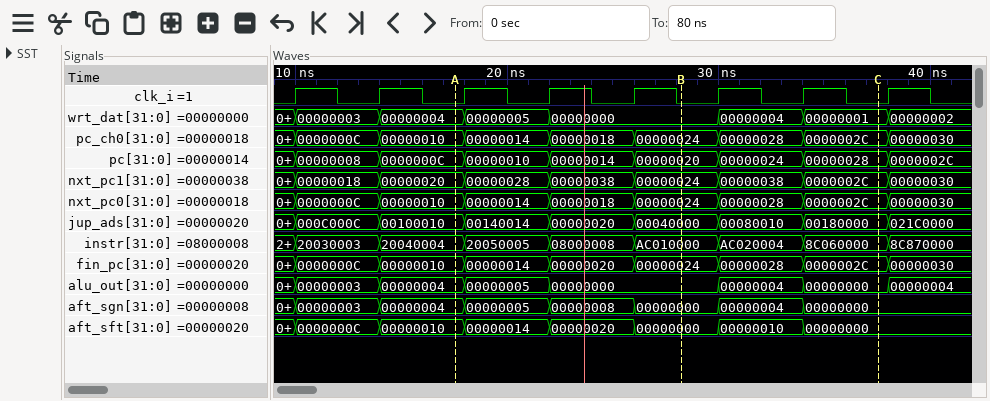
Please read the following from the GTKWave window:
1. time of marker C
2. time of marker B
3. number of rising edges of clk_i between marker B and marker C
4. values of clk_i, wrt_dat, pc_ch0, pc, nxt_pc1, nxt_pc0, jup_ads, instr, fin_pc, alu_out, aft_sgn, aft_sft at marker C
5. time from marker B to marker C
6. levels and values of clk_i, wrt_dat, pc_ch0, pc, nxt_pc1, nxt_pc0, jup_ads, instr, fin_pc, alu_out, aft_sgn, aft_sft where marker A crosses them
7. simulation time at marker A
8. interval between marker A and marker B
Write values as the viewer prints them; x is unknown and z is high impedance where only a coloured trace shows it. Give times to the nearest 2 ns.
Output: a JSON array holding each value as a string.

["38 ns", "28 ns", "2", "clk_i=0, wrt_dat=00000001, pc_ch0=0000002C, pc=00000028, nxt_pc1=0000002C, nxt_pc0=0000002C, jup_ads=00180000, instr=8C060000, fin_pc=0000002C, alu_out=00000000, aft_sgn=00000000, aft_sft=00000000", "10 ns", "clk_i=0, wrt_dat=00000004, pc_ch0=00000010, pc=0000000C, nxt_pc1=00000020, nxt_pc0=00000010, jup_ads=00100010, instr=20040004, fin_pc=00000010, alu_out=00000004, aft_sgn=00000004, aft_sft=00000010", "18 ns", "10 ns"]
